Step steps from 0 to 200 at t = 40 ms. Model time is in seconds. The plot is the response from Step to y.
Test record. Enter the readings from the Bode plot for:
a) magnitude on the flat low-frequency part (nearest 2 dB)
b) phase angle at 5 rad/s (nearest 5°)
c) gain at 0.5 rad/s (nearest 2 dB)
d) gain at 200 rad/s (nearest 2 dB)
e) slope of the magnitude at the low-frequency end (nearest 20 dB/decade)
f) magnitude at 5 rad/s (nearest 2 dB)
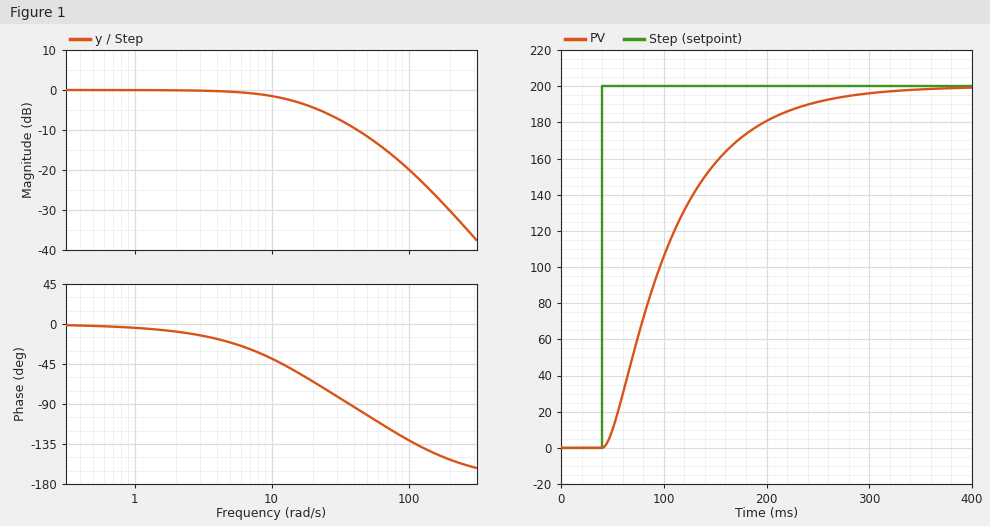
0 dB
-20°
0 dB
-30 dB
0 dB/decade
0 dB
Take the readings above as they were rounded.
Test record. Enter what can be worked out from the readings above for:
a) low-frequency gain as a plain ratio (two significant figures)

1.0
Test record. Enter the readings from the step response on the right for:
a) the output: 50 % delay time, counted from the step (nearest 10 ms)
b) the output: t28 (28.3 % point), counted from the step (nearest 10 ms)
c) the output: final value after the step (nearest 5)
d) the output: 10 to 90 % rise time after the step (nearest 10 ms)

60 ms
30 ms
200
140 ms
